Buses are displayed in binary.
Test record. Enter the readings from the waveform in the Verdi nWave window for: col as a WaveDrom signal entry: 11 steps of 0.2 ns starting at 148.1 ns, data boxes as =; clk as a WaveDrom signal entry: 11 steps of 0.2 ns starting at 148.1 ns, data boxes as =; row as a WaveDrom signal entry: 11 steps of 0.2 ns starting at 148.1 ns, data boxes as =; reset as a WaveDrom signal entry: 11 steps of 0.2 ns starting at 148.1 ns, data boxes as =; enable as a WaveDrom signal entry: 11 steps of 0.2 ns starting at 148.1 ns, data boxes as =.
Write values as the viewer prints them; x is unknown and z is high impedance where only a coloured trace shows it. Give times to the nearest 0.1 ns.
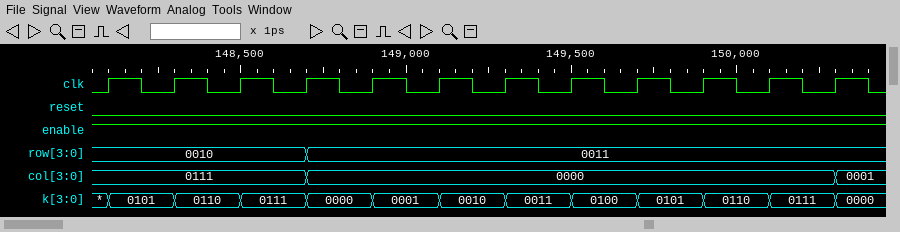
{name: 'col', wave: '=..=.......', data: '0111 0000'}
{name: 'clk', wave: 'p..........'}
{name: 'row', wave: '=..=.......', data: '0010 0011'}
{name: 'reset', wave: '0..........'}
{name: 'enable', wave: '1..........'}
